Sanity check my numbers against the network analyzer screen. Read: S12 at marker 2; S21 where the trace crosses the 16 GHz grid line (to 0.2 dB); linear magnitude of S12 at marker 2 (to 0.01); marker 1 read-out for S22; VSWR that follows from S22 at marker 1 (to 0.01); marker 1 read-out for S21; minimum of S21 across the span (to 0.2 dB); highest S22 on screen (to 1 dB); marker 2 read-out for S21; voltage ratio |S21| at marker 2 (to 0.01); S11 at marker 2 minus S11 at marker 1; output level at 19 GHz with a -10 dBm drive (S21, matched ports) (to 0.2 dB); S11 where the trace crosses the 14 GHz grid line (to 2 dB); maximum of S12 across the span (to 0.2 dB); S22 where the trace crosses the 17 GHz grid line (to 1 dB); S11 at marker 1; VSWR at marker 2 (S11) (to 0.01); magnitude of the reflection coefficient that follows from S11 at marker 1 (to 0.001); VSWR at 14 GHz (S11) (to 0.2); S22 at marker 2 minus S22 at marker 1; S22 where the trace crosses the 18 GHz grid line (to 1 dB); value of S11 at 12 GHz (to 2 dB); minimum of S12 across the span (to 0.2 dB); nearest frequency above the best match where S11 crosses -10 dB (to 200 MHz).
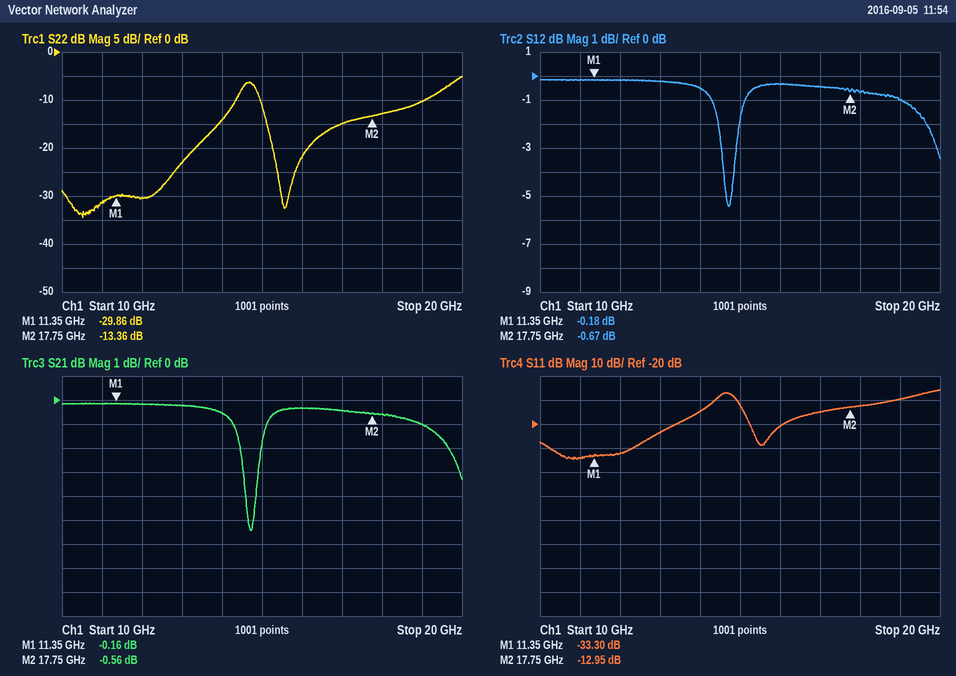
-0.67 dB
-0.4 dB
0.93
-29.86 dB
1.07
-0.16 dB
-5.4 dB
-5 dB
-0.56 dB
0.94
20.35 dB
-11.0 dBm
-14 dB
-0.2 dB
-15 dB
-33.30 dB
1.58
0.022
1.4
16.50 dB
-13 dB
-32 dB
-5.4 dB
14.4 GHz
